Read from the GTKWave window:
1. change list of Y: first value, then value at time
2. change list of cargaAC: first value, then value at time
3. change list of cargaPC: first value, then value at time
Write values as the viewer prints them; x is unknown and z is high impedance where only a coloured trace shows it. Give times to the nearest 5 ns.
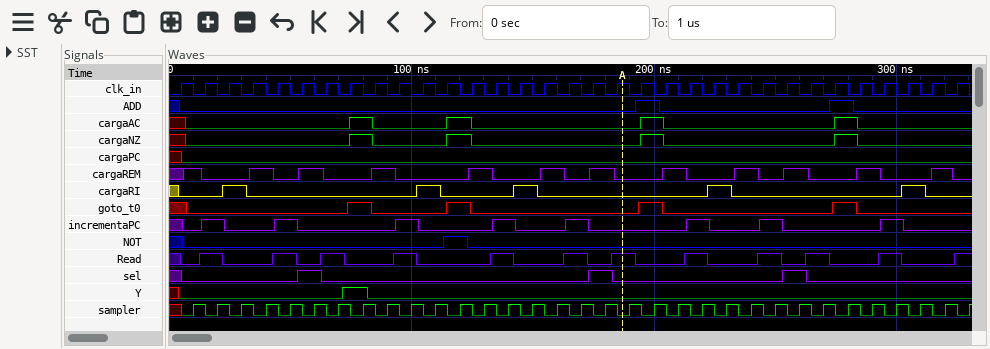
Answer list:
x, 0 at 5 ns, 1 at 70 ns, 0 at 80 ns
x, 0 at 5 ns, 1 at 75 ns, 0 at 85 ns, 1 at 115 ns, 0 at 125 ns, 1 at 195 ns, 0 at 205 ns, 1 at 275 ns, 0 at 285 ns
x, 0 at 5 ns
